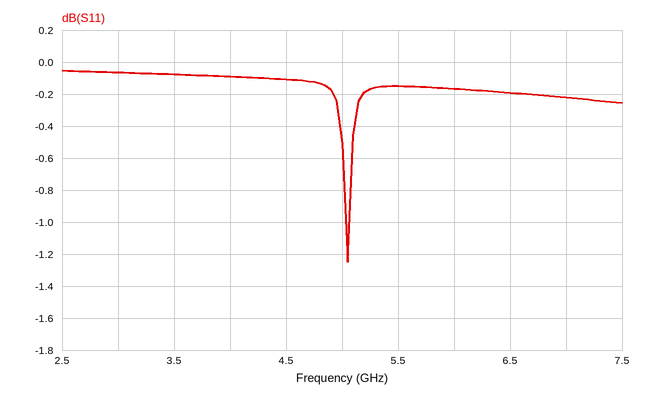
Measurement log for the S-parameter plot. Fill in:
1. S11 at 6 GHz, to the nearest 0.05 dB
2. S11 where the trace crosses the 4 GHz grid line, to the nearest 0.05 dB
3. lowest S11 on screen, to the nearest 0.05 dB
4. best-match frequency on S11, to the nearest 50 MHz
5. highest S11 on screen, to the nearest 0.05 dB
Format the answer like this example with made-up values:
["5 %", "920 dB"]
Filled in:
["-0.15 dB", "-0.10 dB", "-1.25 dB", "5.05 GHz", "-0.05 dB"]
